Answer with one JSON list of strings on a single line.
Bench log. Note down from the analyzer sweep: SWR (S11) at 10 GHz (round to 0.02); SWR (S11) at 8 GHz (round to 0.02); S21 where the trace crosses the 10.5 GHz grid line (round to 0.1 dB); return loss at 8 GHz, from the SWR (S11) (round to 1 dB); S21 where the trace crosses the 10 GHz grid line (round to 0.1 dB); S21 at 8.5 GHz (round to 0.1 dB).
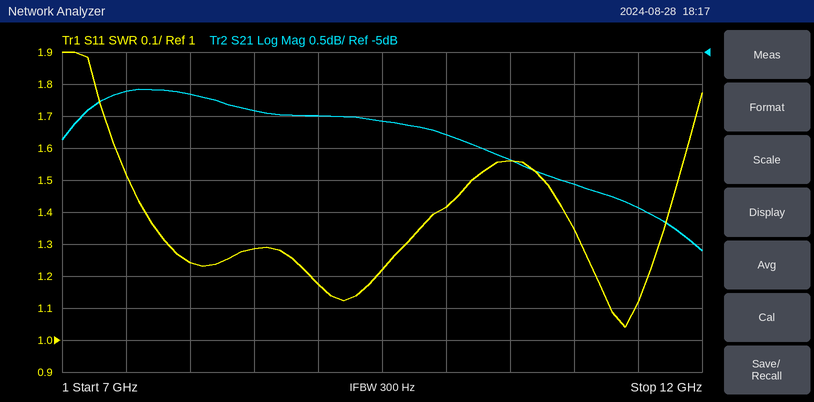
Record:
["1.42", "1.24", "-6.7 dB", "19 dB", "-6.3 dB", "-5.9 dB"]
